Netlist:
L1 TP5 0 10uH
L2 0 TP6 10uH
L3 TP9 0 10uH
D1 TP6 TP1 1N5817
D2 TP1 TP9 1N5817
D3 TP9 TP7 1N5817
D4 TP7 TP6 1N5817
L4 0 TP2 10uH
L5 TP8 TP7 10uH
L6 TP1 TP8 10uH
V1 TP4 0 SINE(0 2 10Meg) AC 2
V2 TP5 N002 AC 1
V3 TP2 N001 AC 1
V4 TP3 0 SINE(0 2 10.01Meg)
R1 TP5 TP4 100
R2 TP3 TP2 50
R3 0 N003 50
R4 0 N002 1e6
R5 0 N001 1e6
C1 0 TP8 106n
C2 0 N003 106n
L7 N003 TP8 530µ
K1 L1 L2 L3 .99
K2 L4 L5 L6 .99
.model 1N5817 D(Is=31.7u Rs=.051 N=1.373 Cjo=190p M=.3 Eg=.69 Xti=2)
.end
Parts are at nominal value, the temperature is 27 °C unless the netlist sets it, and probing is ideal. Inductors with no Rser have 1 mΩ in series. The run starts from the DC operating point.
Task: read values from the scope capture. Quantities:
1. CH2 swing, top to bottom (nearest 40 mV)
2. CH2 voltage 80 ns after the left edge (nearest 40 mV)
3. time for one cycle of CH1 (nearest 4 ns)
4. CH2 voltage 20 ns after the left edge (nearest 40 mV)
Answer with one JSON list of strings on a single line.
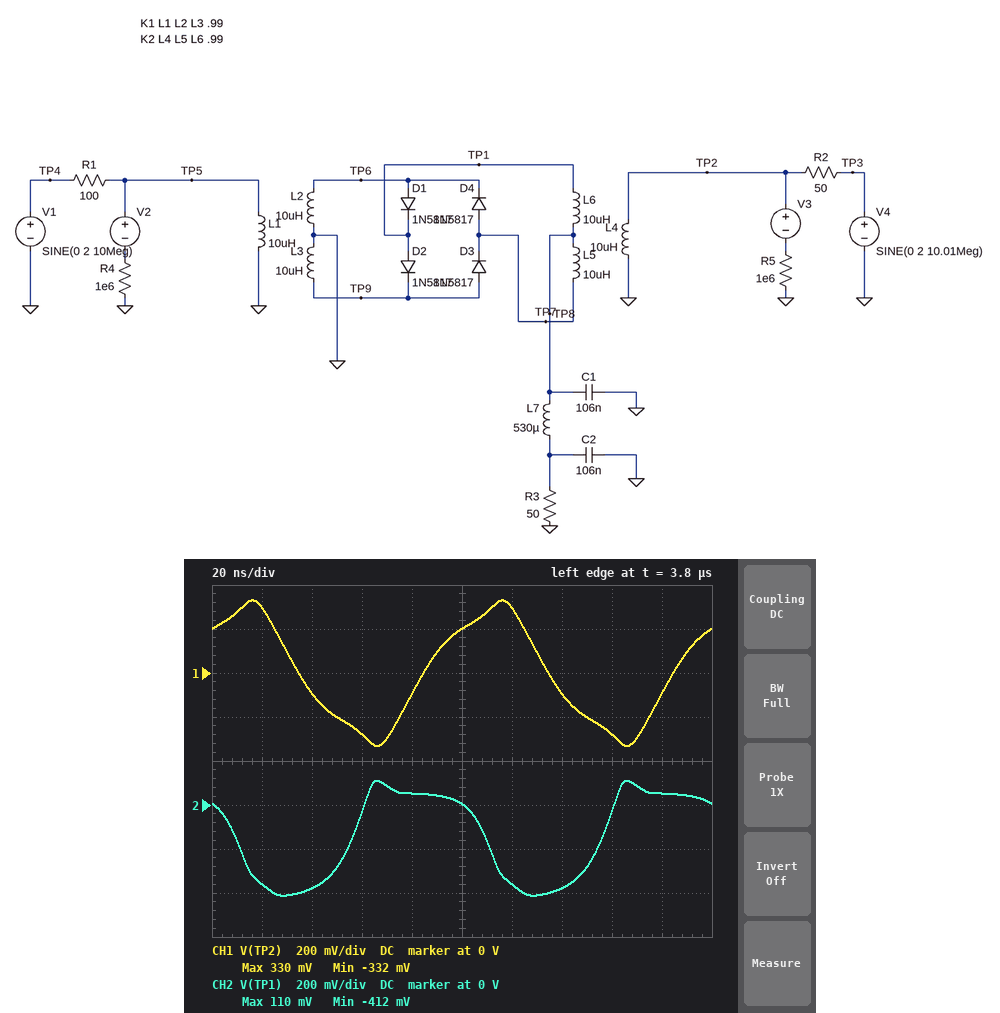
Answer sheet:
["520 mV", "40 mV", "100 ns", "-360 mV"]
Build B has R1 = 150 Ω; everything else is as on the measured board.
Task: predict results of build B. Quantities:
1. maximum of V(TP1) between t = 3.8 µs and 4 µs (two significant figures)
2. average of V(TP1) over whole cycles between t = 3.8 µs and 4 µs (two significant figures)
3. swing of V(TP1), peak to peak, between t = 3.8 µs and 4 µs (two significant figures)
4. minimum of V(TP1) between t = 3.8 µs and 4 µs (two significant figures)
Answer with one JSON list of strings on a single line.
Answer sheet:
["150 mV", "-120 mV", "530 mV", "-380 mV"]
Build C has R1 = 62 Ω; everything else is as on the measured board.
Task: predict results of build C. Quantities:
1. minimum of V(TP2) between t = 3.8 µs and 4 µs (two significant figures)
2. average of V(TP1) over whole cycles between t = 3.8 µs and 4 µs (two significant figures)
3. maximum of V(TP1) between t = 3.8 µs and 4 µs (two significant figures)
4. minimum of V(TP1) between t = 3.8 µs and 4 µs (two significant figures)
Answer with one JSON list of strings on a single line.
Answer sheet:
["-330 mV", "-170 mV", "73 mV", "-430 mV"]
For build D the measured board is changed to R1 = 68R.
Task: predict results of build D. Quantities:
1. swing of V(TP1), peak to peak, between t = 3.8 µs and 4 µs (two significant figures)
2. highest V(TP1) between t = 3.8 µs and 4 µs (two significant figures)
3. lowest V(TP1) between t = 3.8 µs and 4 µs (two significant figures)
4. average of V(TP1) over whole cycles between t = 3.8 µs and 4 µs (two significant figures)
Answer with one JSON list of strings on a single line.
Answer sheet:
["510 mV", "79 mV", "-430 mV", "-160 mV"]
